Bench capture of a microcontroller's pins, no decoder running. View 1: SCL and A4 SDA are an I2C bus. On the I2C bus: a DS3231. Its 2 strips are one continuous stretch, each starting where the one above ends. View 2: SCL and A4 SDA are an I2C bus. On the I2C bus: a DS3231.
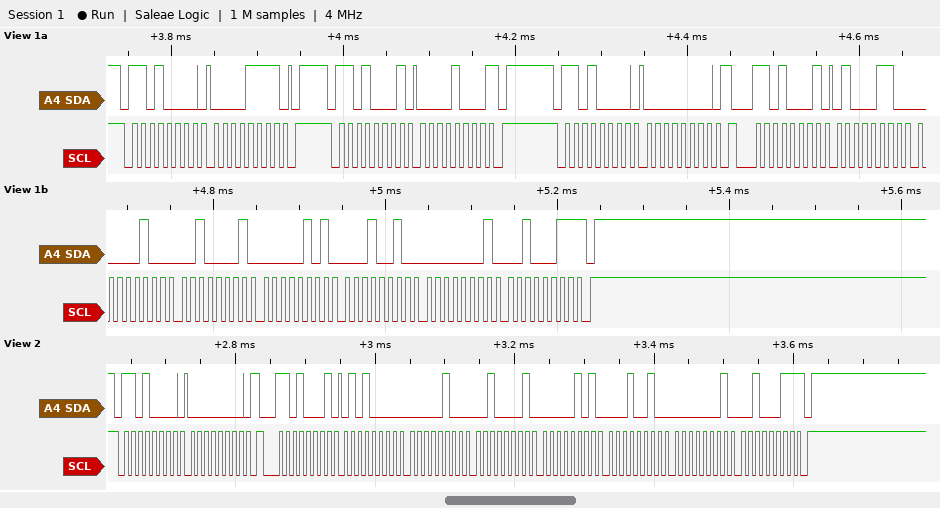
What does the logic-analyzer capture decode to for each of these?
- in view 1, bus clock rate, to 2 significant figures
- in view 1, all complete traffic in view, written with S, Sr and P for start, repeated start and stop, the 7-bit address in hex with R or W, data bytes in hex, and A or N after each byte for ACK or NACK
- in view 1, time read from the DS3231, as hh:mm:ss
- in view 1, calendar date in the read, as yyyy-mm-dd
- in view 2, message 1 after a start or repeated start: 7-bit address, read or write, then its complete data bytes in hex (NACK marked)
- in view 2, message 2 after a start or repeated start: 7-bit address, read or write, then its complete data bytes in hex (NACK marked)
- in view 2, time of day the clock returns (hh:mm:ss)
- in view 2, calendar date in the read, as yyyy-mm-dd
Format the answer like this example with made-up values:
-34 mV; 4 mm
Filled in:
100 kHz; S 68W A 0F A P S 68R A 08 N P S 68W A 00 A Sr 68R A 46 A 04 A 21 A 05 A 12 A 01 A 23 N P; 21:04:46; 2023-01-12; 0x68 write: 00; 0x68 read: 50 04 21 05 12 01 23 NACK; 21:04:50; 2023-01-12
